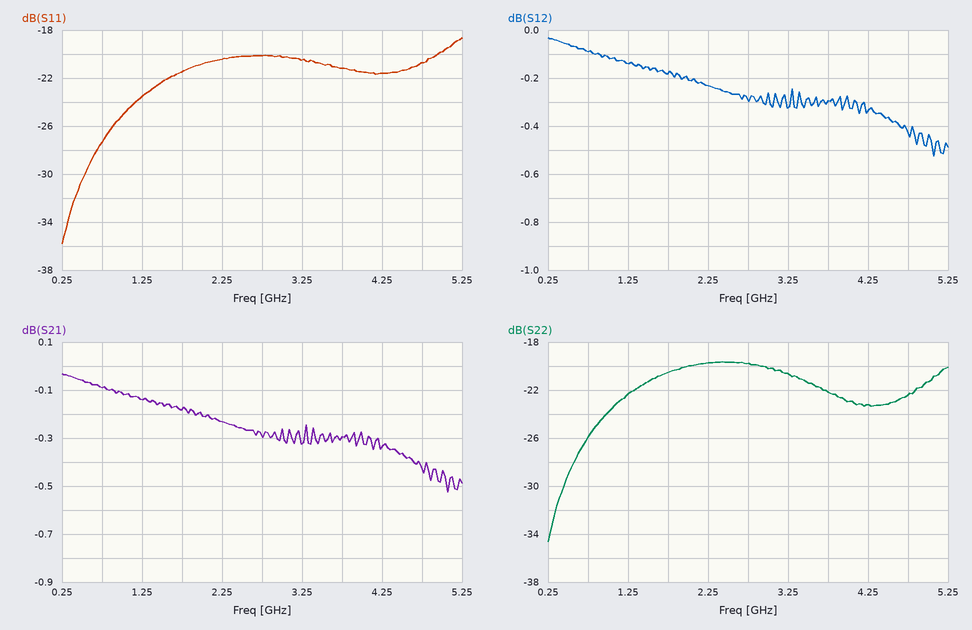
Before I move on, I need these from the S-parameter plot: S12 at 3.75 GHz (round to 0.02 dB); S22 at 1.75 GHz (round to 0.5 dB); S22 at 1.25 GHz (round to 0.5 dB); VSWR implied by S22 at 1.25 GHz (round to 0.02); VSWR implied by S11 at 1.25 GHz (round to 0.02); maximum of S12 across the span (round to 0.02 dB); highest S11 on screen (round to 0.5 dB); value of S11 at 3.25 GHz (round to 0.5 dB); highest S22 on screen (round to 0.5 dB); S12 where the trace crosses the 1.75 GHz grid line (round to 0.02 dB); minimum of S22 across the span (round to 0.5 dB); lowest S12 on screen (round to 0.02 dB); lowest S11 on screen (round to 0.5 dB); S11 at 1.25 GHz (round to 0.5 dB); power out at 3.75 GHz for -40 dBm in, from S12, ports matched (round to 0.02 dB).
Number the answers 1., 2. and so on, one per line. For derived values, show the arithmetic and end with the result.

1. -0.30 dB
2. -20.5 dB
3. -22.5 dB
4. |Γ| = 10^(-22.5/20) = 0.0750; VSWR = (1 + 0.0750)/(1 − 0.0750) ≈ 1.16
5. |Γ| = 10^(-23.5/20) = 0.0668; VSWR = (1 + 0.0668)/(1 − 0.0668) ≈ 1.14
6. -0.04 dB
7. -18.5 dB
8. -20.5 dB
9. -19.5 dB
10. -0.18 dB
11. -34.5 dB
12. -0.52 dB
13. -36.0 dB
14. -23.5 dB
15. -40 dBm + (-0.30 dB) = -40.30 dBm
